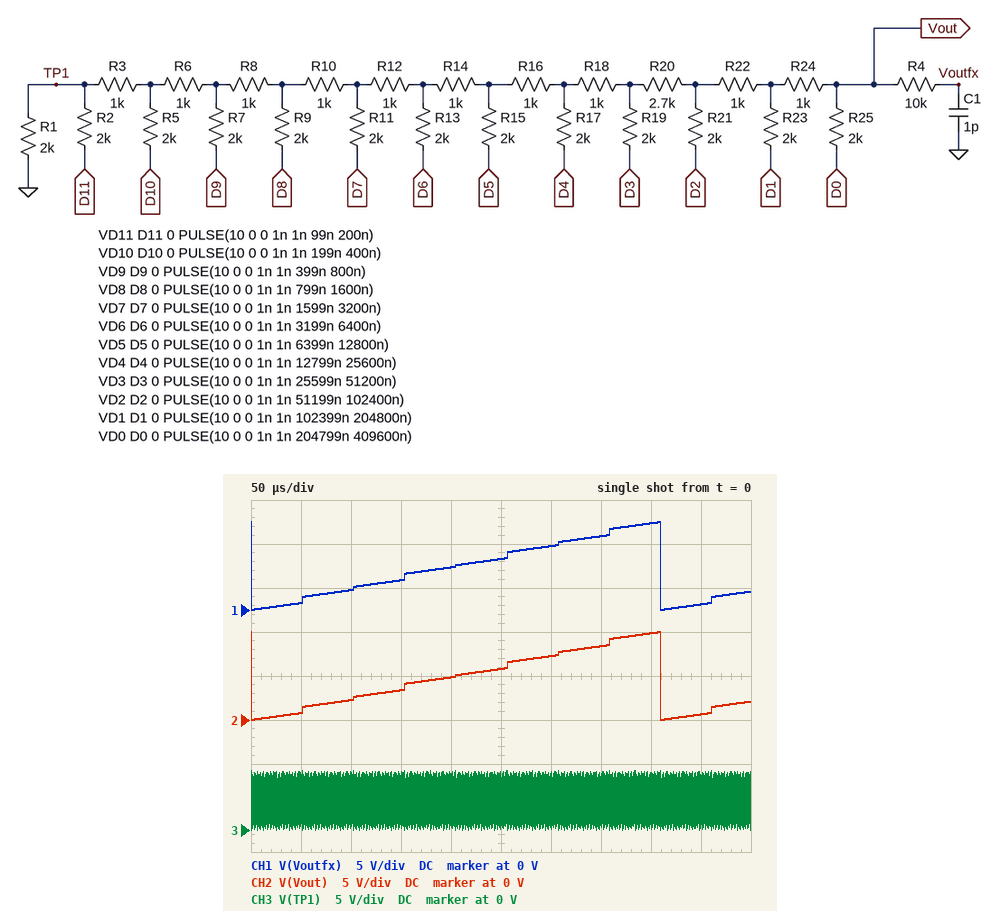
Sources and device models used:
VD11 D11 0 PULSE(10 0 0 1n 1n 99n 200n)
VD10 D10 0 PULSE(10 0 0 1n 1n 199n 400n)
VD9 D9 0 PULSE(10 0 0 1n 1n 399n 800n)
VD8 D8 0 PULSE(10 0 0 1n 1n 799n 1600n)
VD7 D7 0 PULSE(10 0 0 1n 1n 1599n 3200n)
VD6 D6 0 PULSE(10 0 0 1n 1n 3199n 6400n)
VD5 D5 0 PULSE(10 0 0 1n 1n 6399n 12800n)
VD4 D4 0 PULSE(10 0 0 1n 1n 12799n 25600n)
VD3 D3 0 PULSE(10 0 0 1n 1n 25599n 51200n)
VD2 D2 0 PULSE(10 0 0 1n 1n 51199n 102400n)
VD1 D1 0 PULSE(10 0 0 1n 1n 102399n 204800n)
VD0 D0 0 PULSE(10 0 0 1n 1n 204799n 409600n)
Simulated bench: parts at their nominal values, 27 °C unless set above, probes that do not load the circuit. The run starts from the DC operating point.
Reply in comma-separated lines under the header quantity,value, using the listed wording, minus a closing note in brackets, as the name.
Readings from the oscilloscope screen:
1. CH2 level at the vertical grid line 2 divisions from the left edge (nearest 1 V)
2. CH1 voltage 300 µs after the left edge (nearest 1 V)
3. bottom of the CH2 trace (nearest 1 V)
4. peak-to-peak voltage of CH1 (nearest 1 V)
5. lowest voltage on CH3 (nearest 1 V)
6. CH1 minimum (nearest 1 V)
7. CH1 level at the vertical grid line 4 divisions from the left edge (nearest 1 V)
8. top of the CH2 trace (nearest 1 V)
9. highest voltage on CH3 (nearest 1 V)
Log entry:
quantity,value
CH2 level at the vertical grid line 2 divisions from the left edge,2 V
CH1 voltage 300 µs after the left edge,7 V
bottom of the CH2 trace,0 V
peak-to-peak voltage of CH1,10 V
lowest voltage on CH3,0 V
CH1 minimum,0 V
CH1 level at the vertical grid line 4 divisions from the left edge,5 V
top of the CH2 trace,10 V
highest voltage on CH3,7 V
